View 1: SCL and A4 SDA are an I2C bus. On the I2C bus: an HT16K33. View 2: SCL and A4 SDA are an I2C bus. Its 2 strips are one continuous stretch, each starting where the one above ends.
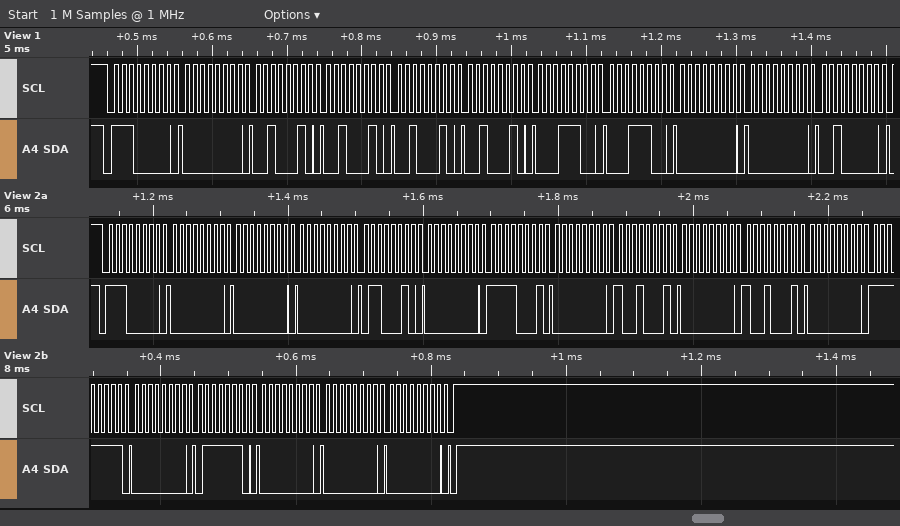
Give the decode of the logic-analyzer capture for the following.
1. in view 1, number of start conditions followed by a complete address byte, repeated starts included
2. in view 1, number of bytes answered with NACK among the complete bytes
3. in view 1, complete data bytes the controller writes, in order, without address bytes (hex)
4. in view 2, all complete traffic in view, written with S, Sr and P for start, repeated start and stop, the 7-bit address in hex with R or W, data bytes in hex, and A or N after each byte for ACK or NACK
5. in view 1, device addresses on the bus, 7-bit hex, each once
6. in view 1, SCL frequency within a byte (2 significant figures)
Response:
1
0
00 22 22 22 22 1C 1C 00 00 20
S 70W A 00 A 00 A 00 A 62 A 00 A F1 A 00 A 91 A 00 A 91 A 00 A FF A 00 A 7E A 00 A 00 A 00 A P
0x70
100 kHz
